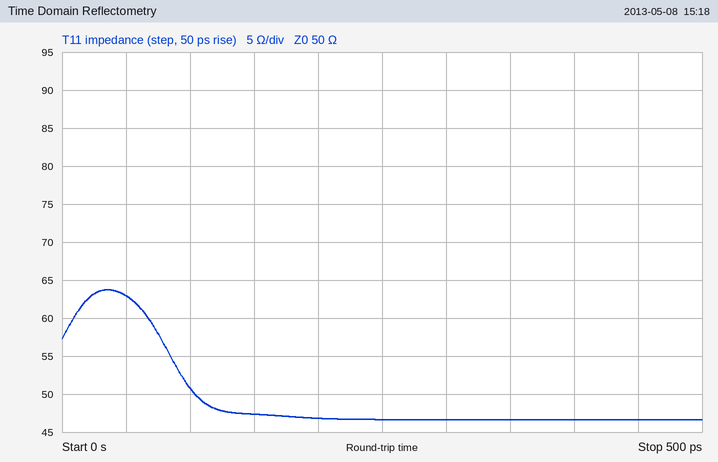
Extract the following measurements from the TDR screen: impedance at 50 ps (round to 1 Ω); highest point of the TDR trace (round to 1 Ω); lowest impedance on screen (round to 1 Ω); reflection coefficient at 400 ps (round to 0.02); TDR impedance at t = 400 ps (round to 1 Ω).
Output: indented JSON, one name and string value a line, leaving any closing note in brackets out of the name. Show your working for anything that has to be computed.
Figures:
{
  "impedance at 50 ps": "63 Ω",
  "highest point of the TDR trace": "64 Ω",
  "lowest impedance on screen": "47 Ω",
  "reflection coefficient at 400 ps": "(47 − 50)/(47 + 50) ≈ -0.0309, so -0.04 to the nearest 0.02",
  "TDR impedance at t = 400 ps": "47 Ω"
}
